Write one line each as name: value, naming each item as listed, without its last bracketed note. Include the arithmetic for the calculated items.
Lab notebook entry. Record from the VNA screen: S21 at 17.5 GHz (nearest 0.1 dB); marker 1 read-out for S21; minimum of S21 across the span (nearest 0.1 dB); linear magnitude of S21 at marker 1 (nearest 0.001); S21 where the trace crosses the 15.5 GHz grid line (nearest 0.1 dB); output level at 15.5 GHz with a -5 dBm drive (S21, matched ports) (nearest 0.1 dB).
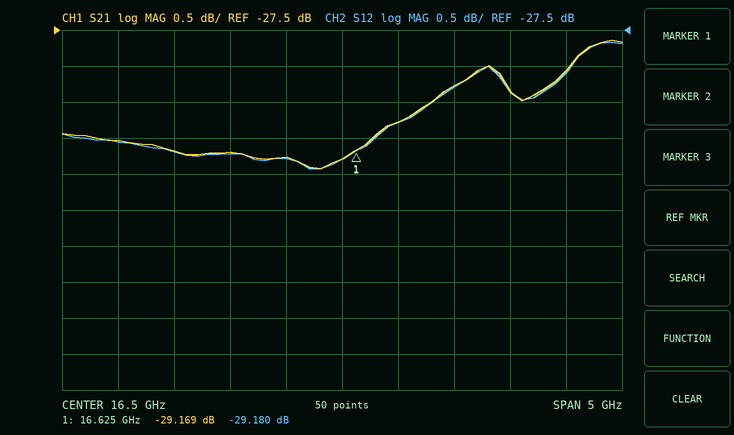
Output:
S21 at 17.5 GHz: -28.3 dB
marker 1 read-out for S21: -29.169 dB
minimum of S21 across the span: -29.4 dB
linear magnitude of S21 at marker 1: 10^(-29.169/20) ≈ 0.035
S21 where the trace crosses the 15.5 GHz grid line: -29.2 dB
output level at 15.5 GHz with a -5 dBm drive (S21, matched ports): -5 dBm + (-29.2 dB) = -34.2 dBm
